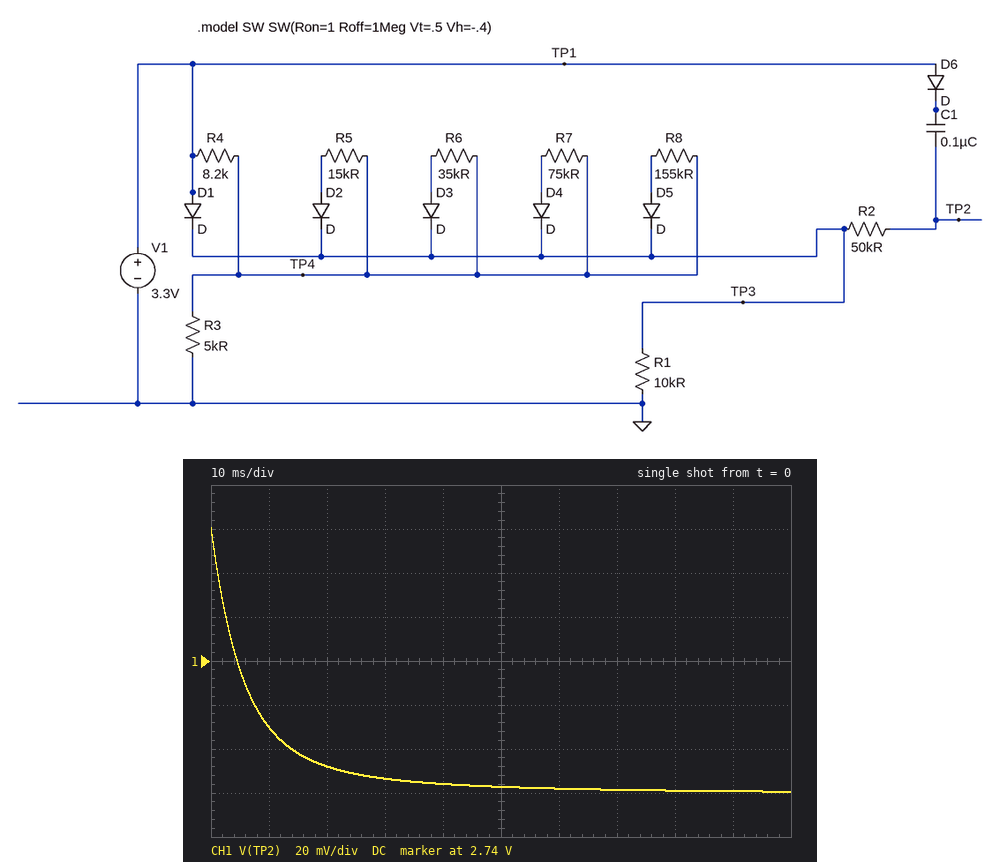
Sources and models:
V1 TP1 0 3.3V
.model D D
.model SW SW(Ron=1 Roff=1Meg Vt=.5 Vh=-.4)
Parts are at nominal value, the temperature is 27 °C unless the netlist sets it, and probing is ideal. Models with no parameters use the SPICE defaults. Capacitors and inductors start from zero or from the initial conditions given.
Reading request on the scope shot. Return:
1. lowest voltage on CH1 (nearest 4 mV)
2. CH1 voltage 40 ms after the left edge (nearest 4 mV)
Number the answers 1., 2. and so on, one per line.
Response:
1. 2.680 V
2. 2.684 V
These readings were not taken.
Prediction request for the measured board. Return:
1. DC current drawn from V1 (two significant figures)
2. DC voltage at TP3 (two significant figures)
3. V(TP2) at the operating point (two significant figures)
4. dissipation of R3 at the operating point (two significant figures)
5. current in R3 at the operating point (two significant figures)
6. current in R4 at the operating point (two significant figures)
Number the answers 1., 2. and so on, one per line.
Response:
1. 520 µA
2. 2.7 V
3. 2.7 V
4. 310 µW
5. 250 µA
6. 250 µA
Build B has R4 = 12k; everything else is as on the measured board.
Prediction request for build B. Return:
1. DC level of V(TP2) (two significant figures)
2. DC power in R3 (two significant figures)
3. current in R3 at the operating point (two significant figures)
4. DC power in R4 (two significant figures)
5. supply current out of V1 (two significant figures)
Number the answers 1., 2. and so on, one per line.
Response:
1. 2.7 V
2. 190 µW
3. 190 µA
4. 450 µW
5. 460 µA
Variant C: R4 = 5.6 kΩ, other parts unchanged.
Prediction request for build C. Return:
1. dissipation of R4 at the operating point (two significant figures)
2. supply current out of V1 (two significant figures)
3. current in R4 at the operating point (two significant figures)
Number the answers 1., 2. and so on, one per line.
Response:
1. 540 µW
2. 580 µA
3. 310 µA
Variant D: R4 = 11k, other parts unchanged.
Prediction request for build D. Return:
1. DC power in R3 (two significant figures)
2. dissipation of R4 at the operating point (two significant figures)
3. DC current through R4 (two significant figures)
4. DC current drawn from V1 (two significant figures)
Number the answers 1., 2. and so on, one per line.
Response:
1. 210 µW
2. 470 µW
3. 210 µA
4. 470 µA
